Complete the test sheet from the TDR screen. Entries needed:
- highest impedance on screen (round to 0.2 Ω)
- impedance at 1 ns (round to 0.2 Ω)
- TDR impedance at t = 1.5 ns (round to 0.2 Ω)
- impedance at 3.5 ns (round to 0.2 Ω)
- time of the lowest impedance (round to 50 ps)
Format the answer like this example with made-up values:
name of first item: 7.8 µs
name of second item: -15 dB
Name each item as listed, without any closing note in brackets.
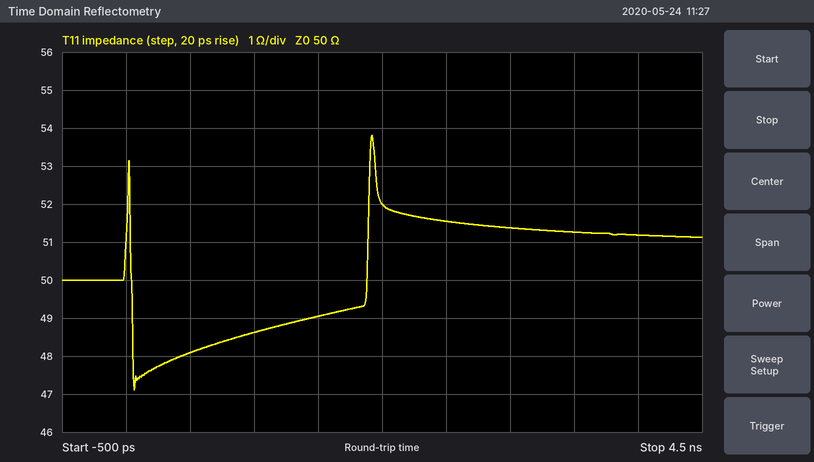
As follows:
highest impedance on screen: 53.8 Ω
impedance at 1 ns: 48.6 Ω
TDR impedance at t = 1.5 ns: 49.0 Ω
impedance at 3.5 ns: 51.2 Ω
time of the lowest impedance: 50 ps
